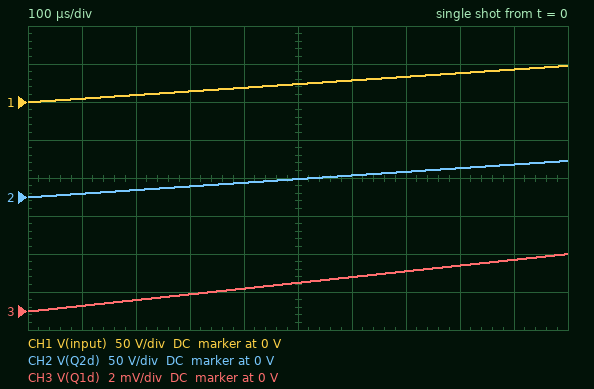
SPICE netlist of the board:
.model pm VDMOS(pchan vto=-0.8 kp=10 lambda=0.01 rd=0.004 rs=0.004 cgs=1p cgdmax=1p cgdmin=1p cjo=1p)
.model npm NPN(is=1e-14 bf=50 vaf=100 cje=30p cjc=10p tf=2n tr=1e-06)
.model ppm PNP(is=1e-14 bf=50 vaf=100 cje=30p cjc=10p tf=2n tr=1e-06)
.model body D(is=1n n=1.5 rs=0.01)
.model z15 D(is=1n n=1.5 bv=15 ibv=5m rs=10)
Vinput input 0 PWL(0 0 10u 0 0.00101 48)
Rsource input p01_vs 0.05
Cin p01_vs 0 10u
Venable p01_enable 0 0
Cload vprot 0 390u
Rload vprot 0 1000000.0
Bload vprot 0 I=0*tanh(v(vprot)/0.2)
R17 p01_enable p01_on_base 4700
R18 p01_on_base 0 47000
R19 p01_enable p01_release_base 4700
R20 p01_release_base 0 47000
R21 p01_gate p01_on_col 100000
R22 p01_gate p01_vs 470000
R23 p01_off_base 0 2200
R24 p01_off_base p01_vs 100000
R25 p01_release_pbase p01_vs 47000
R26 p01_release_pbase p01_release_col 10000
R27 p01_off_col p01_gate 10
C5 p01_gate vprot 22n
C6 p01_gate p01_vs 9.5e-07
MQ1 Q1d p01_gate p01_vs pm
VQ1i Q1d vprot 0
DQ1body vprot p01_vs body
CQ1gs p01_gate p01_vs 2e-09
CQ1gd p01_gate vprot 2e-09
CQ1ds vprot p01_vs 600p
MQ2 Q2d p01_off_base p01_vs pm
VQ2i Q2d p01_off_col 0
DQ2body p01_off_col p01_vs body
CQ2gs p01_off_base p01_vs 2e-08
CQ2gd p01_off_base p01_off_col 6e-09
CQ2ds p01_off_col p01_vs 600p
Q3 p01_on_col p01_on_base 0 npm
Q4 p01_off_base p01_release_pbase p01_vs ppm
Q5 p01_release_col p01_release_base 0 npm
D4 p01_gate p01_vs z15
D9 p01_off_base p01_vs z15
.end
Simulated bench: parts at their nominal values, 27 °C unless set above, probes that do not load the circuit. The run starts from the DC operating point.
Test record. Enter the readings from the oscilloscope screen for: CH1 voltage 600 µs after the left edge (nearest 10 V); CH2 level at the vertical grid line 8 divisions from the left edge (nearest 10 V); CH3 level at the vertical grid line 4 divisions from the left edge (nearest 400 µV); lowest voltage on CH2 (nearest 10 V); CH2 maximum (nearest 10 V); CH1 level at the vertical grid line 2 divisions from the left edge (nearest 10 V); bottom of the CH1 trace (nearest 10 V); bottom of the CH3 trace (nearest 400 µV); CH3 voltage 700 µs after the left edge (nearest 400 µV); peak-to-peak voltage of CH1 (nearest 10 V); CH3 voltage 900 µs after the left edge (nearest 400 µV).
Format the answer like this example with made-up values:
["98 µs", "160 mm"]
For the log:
["30 V", "40 V", "1.2 mV", "0 V", "50 V", "10 V", "0 V", "0 V", "2.0 mV", "50 V", "2.8 mV"]
